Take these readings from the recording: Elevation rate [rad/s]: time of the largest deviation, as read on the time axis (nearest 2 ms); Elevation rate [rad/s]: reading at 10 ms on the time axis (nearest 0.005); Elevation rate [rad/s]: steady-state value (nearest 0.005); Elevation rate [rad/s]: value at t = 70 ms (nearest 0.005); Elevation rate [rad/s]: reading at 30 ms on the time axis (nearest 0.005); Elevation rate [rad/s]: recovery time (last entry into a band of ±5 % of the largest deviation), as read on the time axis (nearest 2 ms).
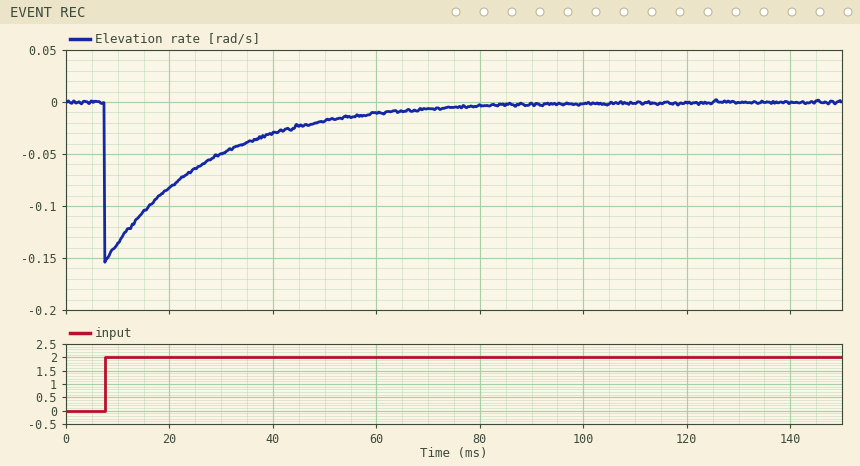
8 ms
-0.135
0.000
-0.005
-0.050
68 ms
